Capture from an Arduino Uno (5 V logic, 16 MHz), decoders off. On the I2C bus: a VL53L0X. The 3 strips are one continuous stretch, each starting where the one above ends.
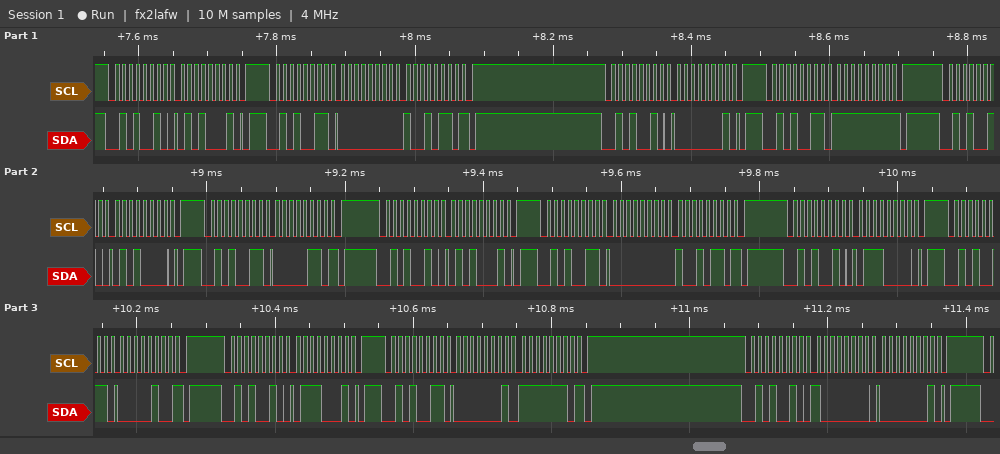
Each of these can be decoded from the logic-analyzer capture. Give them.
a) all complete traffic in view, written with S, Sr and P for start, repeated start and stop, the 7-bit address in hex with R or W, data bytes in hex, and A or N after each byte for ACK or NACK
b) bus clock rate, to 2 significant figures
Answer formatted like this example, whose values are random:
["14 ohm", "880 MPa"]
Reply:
["S 29W A 51 A P S 29R A 00 A 96 N P S 29W A 01 A P S 29R A FF N P S 29W A 50 A P S 29R A 06 N P S 29W A 51 A P S 29R A 00 A 96 N P S 29W A 70 A P S 29R A 04 N P S 29W A 71 A P S 29R A 01 A FE N P S 29W A 80 A 01 A P", "100 kHz"]
